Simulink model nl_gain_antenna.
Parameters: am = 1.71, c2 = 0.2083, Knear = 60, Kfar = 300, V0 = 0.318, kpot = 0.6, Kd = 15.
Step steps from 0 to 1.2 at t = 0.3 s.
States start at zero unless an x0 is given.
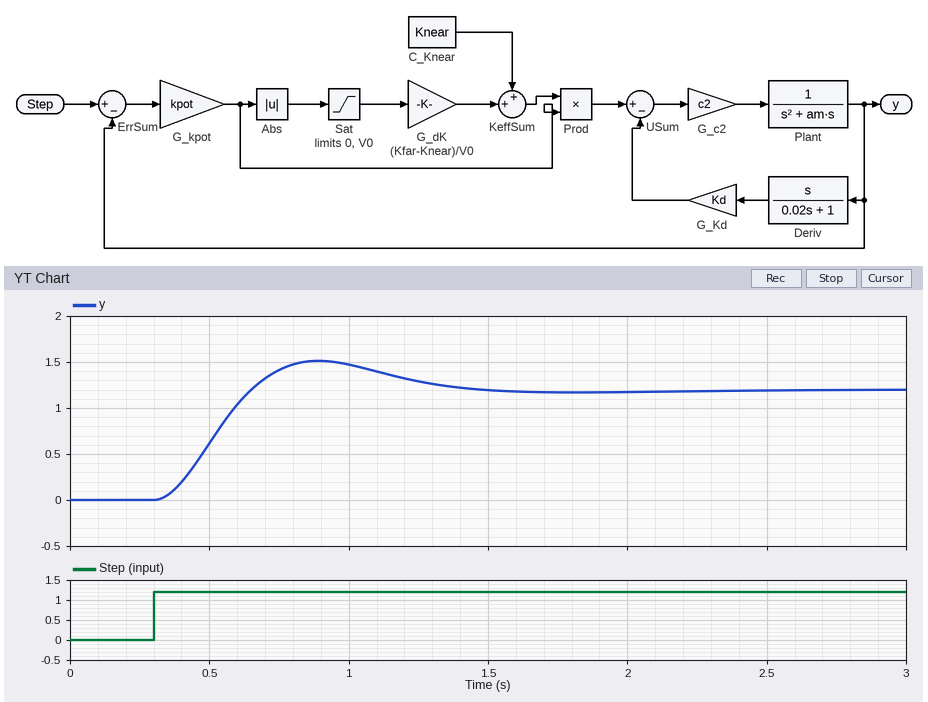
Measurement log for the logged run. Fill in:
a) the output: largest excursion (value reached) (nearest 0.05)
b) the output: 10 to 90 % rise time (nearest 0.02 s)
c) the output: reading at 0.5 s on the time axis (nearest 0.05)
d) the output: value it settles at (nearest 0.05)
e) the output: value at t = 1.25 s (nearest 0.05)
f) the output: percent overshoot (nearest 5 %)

1.50
0.24 s
0.60
1.20
1.30
25 %
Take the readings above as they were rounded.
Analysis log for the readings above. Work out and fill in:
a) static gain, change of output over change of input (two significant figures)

1.0
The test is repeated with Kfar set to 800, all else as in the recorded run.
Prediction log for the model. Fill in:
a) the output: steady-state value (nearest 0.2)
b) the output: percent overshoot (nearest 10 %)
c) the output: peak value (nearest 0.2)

1.2
50 %
1.8
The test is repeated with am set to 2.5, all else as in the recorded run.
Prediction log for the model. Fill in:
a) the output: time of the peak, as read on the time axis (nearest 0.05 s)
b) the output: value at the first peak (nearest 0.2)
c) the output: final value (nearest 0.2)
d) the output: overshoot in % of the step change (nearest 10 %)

0.95 s
1.4
1.2
20 %
